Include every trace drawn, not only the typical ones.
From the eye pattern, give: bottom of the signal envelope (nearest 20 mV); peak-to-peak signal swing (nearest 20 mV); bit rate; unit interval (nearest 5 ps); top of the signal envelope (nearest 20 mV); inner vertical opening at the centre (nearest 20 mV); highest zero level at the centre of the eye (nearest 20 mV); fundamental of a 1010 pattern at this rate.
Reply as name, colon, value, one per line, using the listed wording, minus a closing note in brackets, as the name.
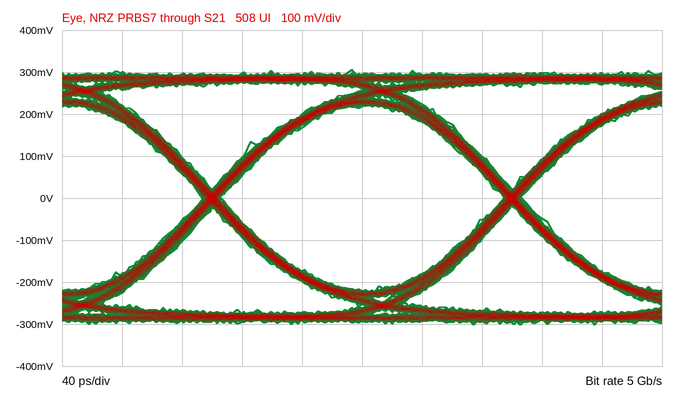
bottom of the signal envelope: -300 mV
peak-to-peak signal swing: 600 mV
bit rate: 5 Gb/s
unit interval: 200 ps
top of the signal envelope: 300 mV
inner vertical opening at the centre: 440 mV
highest zero level at the centre of the eye: -220 mV
fundamental of a 1010 pattern at this rate: 2.5 GHz
